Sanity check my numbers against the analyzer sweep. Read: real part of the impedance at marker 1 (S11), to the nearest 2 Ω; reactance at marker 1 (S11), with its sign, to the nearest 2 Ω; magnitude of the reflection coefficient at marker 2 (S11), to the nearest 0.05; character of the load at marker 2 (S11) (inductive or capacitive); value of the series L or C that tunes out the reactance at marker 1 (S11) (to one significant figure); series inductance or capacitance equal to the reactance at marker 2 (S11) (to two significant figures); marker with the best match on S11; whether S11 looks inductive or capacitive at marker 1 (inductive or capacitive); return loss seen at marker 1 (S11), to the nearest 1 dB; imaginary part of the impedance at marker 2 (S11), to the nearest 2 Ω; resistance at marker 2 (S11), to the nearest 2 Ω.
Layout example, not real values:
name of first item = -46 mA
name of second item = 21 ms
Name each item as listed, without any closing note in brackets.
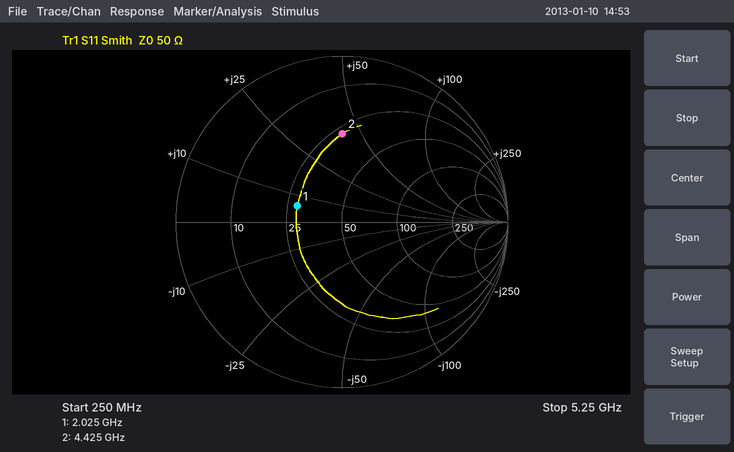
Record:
real part of the impedance at marker 1 (S11), to the nearest 2 Ω = 28 Ω
reactance at marker 1 (S11), with its sign, to the nearest 2 Ω = +6 Ω
magnitude of the reflection coefficient at marker 2 (S11), to the nearest 0.05 = 0.55
character of the load at marker 2 (S11) = inductive
value of the series L or C that tunes out the reactance at marker 1 (S11) = 10 pF
series inductance or capacitance equal to the reactance at marker 2 (S11) = 1.5 nH
marker with the best match on S11 = marker 1
whether S11 looks inductive or capacitive at marker 1 = inductive
return loss seen at marker 1 (S11), to the nearest 1 dB = 11 dB
imaginary part of the impedance at marker 2 (S11), to the nearest 2 Ω = +42 Ω
resistance at marker 2 (S11), to the nearest 2 Ω = 28 Ω
